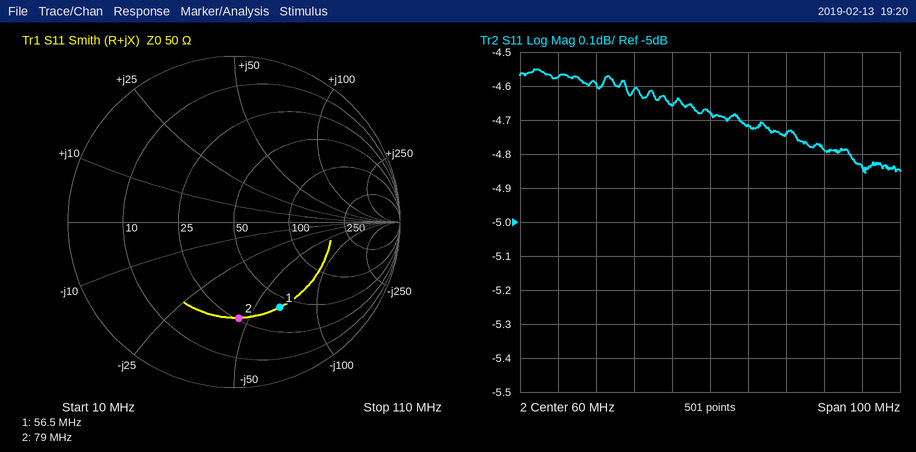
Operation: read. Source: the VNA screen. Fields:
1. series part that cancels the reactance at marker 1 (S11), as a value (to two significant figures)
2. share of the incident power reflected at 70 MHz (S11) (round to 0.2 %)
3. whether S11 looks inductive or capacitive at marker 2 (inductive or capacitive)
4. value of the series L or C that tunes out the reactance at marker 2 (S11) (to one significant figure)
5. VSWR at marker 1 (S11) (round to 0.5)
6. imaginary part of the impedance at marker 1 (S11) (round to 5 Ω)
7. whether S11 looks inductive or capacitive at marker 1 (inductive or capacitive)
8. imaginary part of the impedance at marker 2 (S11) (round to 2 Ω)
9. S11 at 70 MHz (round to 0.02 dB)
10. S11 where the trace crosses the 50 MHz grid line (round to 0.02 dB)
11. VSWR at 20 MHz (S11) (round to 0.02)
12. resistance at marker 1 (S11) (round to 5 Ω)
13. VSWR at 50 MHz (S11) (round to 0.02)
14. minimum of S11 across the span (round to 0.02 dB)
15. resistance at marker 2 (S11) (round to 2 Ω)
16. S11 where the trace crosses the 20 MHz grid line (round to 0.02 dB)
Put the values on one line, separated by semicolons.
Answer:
180 nH; 33.8 %; capacitive; 90 nH; 4.0; -65 Ω; capacitive; -46 Ω; -4.72 dB; -4.66 dB; 3.88; 40 Ω; 3.82; -4.86 dB; 26 Ω; -4.58 dB
